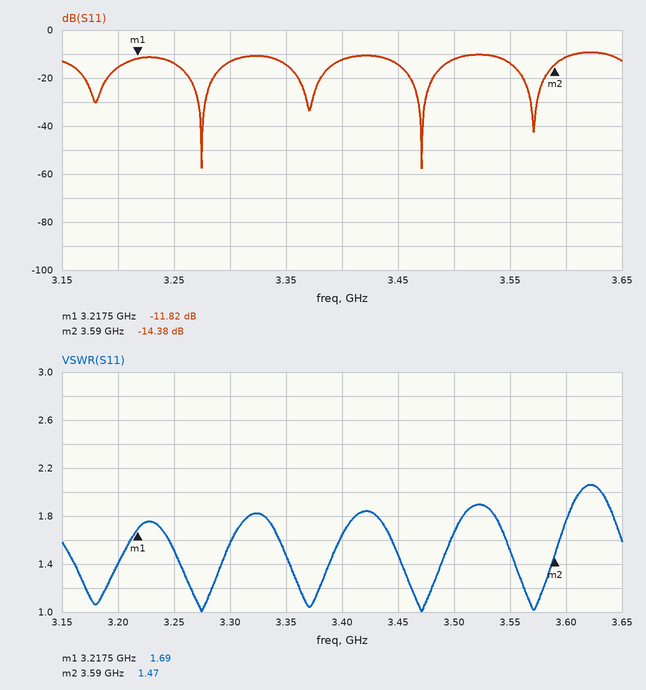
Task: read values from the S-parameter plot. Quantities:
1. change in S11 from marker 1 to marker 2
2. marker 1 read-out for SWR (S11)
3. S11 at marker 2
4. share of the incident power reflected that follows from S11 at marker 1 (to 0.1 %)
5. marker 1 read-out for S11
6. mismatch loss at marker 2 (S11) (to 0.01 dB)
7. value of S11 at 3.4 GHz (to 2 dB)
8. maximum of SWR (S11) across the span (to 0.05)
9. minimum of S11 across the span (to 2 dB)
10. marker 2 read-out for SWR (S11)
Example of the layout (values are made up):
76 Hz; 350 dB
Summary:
-2.56 dB; 1.69; -14.38 dB; 6.6 %; -11.82 dB; 0.16 dB; -12 dB; 2.05; -58 dB; 1.47
